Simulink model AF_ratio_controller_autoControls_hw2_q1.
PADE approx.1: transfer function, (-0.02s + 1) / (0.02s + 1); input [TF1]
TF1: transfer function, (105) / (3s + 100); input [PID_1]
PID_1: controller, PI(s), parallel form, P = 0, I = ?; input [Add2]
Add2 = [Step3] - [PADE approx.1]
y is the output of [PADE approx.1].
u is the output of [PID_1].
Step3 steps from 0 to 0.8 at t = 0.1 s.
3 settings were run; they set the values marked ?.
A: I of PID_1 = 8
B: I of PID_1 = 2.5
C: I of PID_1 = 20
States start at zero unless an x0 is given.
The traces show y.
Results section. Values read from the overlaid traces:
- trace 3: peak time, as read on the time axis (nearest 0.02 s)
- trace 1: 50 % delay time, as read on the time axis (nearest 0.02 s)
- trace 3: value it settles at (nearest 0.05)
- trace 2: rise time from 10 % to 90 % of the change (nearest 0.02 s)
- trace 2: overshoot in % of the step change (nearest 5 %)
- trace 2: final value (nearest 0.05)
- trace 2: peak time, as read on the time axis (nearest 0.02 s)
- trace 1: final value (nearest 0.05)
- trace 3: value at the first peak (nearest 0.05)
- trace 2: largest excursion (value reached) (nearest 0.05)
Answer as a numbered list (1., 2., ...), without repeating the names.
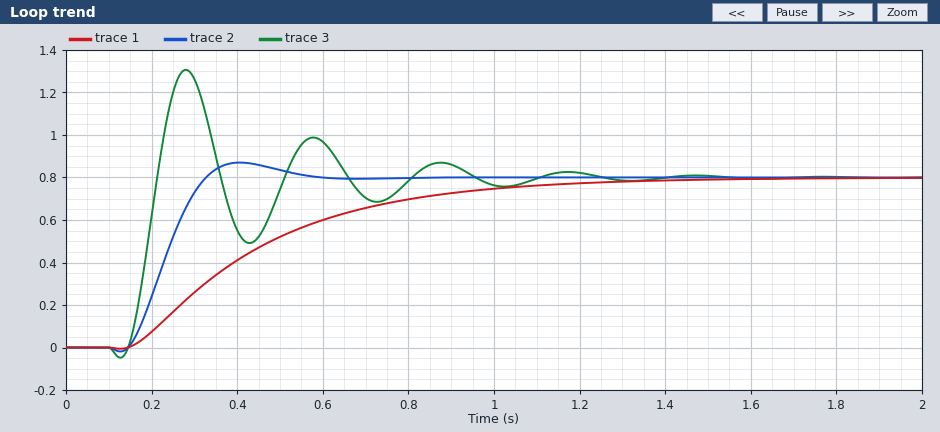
1. 0.28 s
2. 0.40 s
3. 0.80
4. 0.12 s
5. 10 %
6. 0.80
7. 0.40 s
8. 0.80
9. 1.30
10. 0.85
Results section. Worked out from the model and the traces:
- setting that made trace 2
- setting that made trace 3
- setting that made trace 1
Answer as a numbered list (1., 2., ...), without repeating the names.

1. A
2. C
3. B
